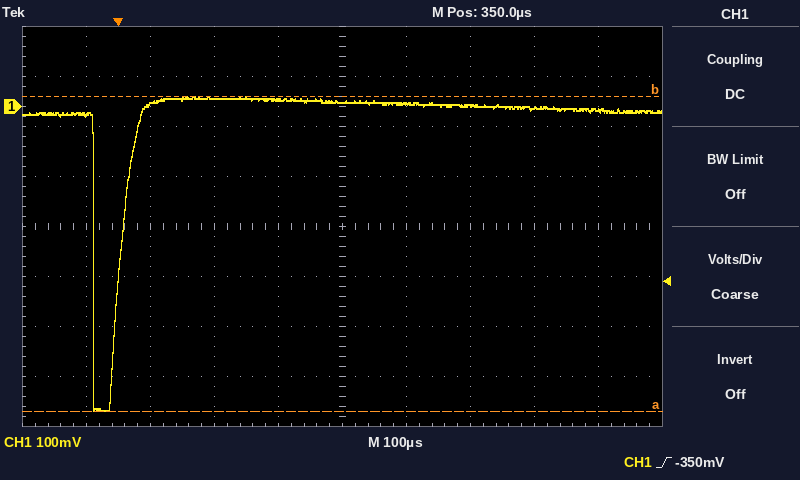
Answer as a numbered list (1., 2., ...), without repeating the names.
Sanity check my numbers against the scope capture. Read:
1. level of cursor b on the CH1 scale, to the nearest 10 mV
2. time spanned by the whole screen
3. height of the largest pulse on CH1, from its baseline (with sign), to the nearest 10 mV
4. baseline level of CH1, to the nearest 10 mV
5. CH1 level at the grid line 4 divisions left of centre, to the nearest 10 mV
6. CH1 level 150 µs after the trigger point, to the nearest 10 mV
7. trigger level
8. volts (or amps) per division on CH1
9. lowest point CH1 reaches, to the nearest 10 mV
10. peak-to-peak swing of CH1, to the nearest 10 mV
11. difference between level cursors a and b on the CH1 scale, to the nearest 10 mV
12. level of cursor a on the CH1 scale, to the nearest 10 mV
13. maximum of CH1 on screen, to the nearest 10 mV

1. 20 mV
2. 1 ms
3. -610 mV
4. 0 mV
5. -20 mV
6. 20 mV
7. -350 mV
8. 100 mV
9. -610 mV
10. 630 mV
11. 630 mV
12. -610 mV
13. 20 mV
